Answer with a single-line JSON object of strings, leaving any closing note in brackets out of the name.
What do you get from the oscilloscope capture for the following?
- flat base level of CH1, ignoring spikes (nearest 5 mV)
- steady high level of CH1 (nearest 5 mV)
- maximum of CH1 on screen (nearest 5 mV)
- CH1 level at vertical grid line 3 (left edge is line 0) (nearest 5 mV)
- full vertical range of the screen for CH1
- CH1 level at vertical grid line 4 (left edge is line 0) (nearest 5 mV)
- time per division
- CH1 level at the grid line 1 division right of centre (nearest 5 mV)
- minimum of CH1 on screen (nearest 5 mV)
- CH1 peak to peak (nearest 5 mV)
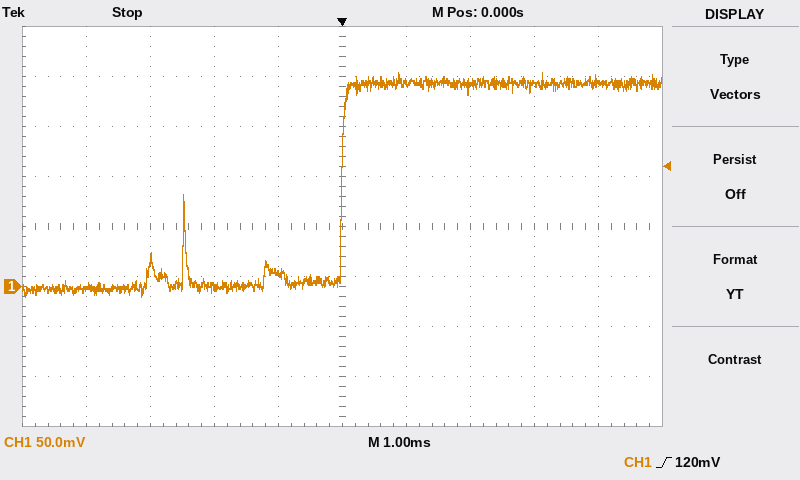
{"flat base level of CH1, ignoring spikes": "0 mV", "steady high level of CH1": "205 mV", "maximum of CH1 on screen": "215 mV", "CH1 level at vertical grid line 3 (left edge is line 0)": "0 mV", "full vertical range of the screen for CH1": "400 mV", "CH1 level at vertical grid line 4 (left edge is line 0)": "15 mV", "time per division": "1 ms", "CH1 level at the grid line 1 division right of centre": "205 mV", "minimum of CH1 on screen": "-10 mV", "CH1 peak to peak": "225 mV"}
